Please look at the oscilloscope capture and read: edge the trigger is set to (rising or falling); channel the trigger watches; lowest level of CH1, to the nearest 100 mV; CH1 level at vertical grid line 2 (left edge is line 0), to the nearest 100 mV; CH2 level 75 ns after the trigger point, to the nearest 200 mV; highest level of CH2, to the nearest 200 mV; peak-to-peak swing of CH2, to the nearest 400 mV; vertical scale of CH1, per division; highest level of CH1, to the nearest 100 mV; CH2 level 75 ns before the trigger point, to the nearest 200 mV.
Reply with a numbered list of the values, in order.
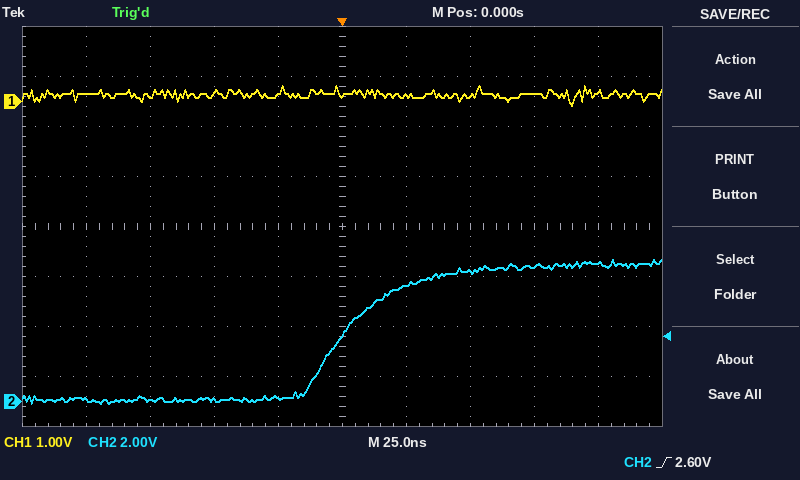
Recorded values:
1. rising
2. CH2
3. -100 mV
4. 100 mV
5. 5.4 V
6. 5.6 V
7. 5.6 V
8. 1 V
9. 300 mV
10. 0.0 V
